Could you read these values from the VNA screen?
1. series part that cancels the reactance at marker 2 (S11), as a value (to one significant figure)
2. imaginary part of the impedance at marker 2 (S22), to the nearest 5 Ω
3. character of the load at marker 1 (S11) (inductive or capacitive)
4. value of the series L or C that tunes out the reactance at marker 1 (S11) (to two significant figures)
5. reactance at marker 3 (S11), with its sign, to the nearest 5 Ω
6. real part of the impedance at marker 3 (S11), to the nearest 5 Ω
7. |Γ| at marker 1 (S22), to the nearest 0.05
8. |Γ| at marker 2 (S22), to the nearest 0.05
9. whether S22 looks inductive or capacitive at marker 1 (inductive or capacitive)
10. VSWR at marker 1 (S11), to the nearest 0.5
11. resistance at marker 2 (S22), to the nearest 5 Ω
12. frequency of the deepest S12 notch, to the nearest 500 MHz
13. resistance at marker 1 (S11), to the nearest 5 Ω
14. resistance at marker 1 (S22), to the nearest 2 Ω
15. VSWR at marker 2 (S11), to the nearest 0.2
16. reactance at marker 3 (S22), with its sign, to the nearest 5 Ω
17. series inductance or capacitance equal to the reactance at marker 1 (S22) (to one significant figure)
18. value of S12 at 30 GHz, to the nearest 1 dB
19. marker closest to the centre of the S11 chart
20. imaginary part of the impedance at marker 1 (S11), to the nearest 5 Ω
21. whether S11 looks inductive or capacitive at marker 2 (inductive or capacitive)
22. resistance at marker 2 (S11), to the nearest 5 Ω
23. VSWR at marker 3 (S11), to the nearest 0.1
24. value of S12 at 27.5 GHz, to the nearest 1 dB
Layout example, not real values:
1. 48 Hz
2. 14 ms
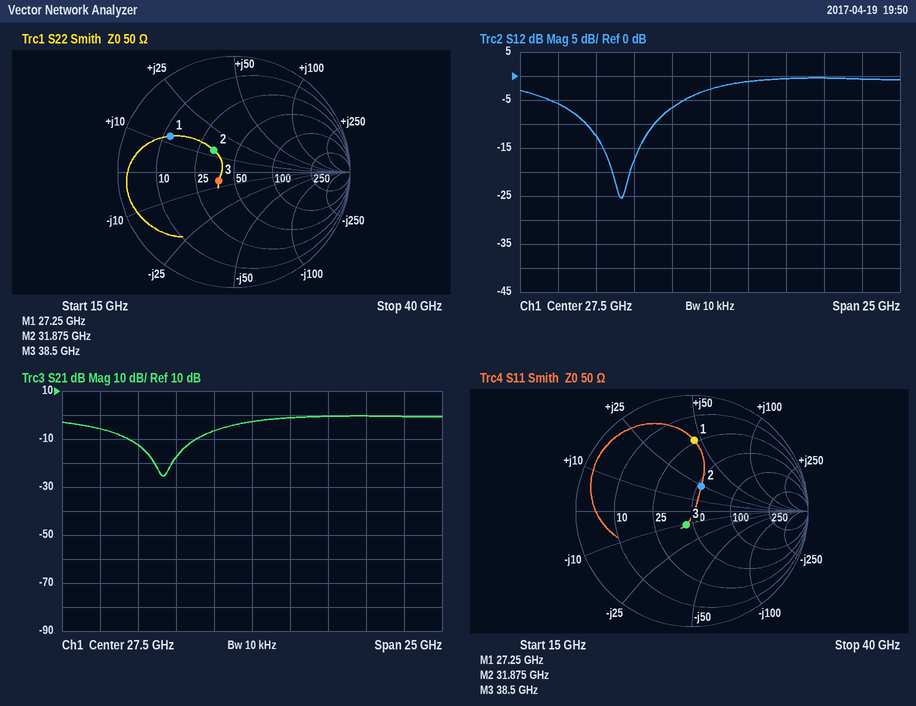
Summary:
1. 200 fF
2. +15 Ω
3. inductive
4. 130 fF
5. -10 Ω
6. 45 Ω
7. 0.65
8. 0.25
9. inductive
10. 4.0
11. 35 Ω
12. 21.5 GHz
13. 25 Ω
14. 12 Ω
15. 1.6
16. -5 Ω
17. 70 pH
18. -1 dB
19. marker 3
20. +45 Ω
21. inductive
22. 55 Ω
23. 1.3
24. -3 dB
